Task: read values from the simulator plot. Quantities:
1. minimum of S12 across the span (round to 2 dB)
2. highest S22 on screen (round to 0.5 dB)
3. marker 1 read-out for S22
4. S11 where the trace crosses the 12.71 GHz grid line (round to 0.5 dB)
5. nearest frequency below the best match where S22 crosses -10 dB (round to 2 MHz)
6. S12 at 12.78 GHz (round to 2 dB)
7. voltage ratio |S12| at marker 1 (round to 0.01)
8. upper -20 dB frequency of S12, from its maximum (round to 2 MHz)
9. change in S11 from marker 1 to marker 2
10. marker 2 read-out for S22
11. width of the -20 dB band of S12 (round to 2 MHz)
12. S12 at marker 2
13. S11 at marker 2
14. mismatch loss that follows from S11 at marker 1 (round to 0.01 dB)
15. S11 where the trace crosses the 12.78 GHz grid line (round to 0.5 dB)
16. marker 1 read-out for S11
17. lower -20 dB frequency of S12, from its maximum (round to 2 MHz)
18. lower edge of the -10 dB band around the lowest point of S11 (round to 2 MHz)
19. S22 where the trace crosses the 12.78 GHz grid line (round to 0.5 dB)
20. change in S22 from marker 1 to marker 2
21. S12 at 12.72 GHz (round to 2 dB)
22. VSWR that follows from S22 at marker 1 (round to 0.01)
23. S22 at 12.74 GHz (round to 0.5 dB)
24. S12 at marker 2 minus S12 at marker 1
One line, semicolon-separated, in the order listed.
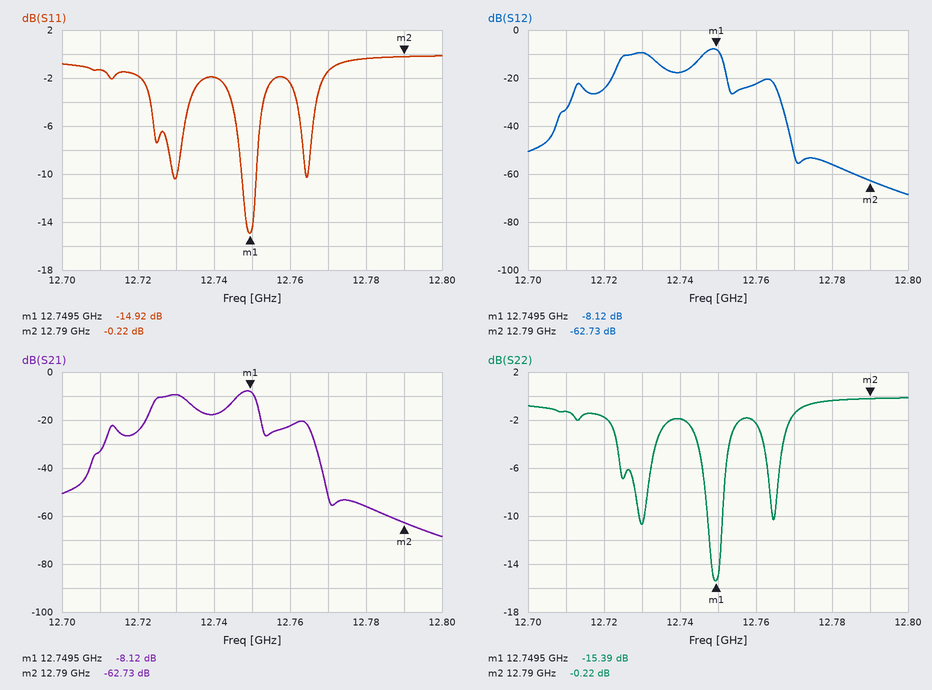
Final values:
-68 dB; 0.0 dB; -15.39 dB; -1.5 dB; 12.748 GHz; -56 dB; 0.39; 12.766 GHz; 14.70 dB; -0.22 dB; 54 MHz; -62.73 dB; -0.22 dB; 0.14 dB; -0.5 dB; -14.92 dB; 12.712 GHz; 12.748 GHz; -0.5 dB; 15.17 dB; -24 dB; 1.41; -2.0 dB; -54.61 dB
